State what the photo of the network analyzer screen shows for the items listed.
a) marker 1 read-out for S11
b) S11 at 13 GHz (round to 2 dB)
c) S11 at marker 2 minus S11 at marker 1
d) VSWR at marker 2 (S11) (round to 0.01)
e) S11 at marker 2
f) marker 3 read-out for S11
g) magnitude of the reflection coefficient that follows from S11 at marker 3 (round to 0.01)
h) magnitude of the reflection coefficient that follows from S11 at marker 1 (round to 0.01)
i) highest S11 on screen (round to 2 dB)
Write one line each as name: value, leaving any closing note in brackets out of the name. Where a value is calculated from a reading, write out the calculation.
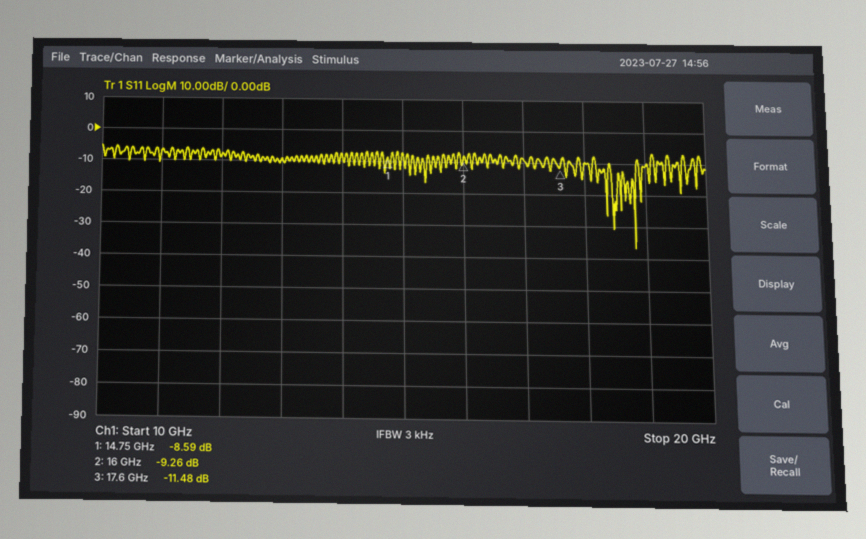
marker 1 read-out for S11: -8.59 dB
S11 at 13 GHz: -10 dB
S11 at marker 2 minus S11 at marker 1: -9.26 − (-8.59) = -0.67 dB
VSWR at marker 2 (S11): (1 + 0.3443)/(1 − 0.3443) ≈ 2.05
S11 at marker 2: -9.26 dB
marker 3 read-out for S11: -11.48 dB
magnitude of the reflection coefficient that follows from S11 at marker 3: 10^(-11.48/20) ≈ 0.27
magnitude of the reflection coefficient that follows from S11 at marker 1: 10^(-8.59/20) ≈ 0.37
highest S11 on screen: -6 dB
